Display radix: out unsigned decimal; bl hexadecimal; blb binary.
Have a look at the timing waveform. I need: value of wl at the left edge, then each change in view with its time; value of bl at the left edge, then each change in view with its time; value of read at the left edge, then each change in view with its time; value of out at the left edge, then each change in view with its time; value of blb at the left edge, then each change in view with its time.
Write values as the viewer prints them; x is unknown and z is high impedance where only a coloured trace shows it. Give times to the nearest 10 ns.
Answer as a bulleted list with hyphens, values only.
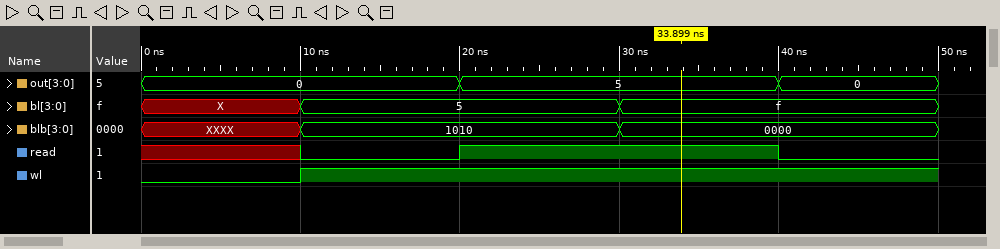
- 0, 1 at 10 ns
- X, 5 at 10 ns, f at 30 ns
- x, 0 at 10 ns, 1 at 20 ns, 0 at 40 ns
- 0, 5 at 20 ns, 0 at 40 ns
- XXXX, 1010 at 10 ns, 0000 at 30 ns
